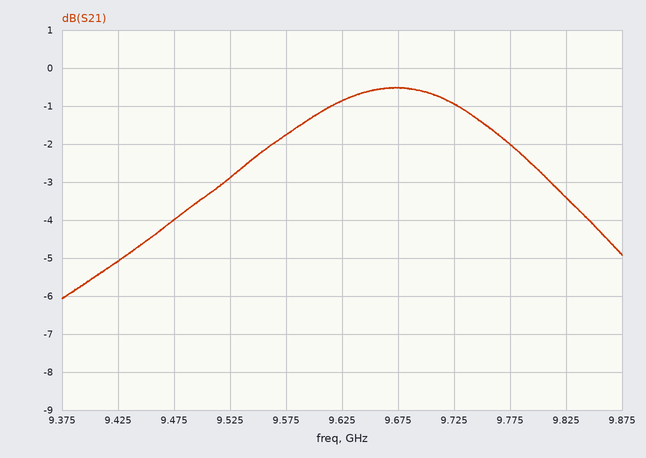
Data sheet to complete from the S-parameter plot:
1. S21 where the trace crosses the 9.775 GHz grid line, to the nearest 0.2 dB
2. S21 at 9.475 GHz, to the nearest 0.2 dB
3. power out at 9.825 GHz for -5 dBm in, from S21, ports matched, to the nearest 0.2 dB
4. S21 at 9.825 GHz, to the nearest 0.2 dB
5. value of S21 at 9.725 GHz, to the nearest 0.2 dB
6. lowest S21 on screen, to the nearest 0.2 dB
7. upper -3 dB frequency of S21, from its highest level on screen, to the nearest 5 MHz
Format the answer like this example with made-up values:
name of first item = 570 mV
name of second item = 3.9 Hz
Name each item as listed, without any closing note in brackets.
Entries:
S21 where the trace crosses the 9.775 GHz grid line, to the nearest 0.2 dB = -2.0 dB
S21 at 9.475 GHz, to the nearest 0.2 dB = -4.0 dB
power out at 9.825 GHz for -5 dBm in, from S21, ports matched, to the nearest 0.2 dB = -8.4 dBm
S21 at 9.825 GHz, to the nearest 0.2 dB = -3.4 dB
value of S21 at 9.725 GHz, to the nearest 0.2 dB = -1.0 dB
lowest S21 on screen, to the nearest 0.2 dB = -6.0 dB
upper -3 dB frequency of S21, from its highest level on screen, to the nearest 5 MHz = 9.830 GHz
